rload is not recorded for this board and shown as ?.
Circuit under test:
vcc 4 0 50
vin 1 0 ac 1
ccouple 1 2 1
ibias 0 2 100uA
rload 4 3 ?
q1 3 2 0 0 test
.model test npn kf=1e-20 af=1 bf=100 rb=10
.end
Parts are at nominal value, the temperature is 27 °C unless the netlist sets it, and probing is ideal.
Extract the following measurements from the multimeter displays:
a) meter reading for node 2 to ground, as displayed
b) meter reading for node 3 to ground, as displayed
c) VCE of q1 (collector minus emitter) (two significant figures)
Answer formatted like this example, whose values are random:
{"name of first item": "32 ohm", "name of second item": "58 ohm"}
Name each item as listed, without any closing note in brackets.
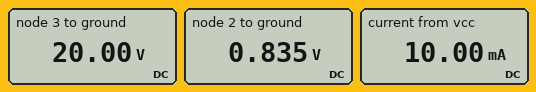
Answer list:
{"meter reading for node 2 to ground, as displayed": "0.835 V", "meter reading for node 3 to ground, as displayed": "20.00 V", "VCE of q1 (collector minus emitter)": "20 V"}
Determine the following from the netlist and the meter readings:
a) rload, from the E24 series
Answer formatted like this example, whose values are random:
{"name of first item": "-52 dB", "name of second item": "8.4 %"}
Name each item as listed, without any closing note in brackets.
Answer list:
{"rload, from the E24 series": "3 kΩ"}
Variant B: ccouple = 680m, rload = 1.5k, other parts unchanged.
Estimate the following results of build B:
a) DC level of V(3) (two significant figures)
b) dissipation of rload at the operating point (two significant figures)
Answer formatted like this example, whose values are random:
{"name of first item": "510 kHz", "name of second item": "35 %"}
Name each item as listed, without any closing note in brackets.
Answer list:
{"DC level of V(3)": "35 V", "dissipation of rload at the operating point": "150 mW"}
